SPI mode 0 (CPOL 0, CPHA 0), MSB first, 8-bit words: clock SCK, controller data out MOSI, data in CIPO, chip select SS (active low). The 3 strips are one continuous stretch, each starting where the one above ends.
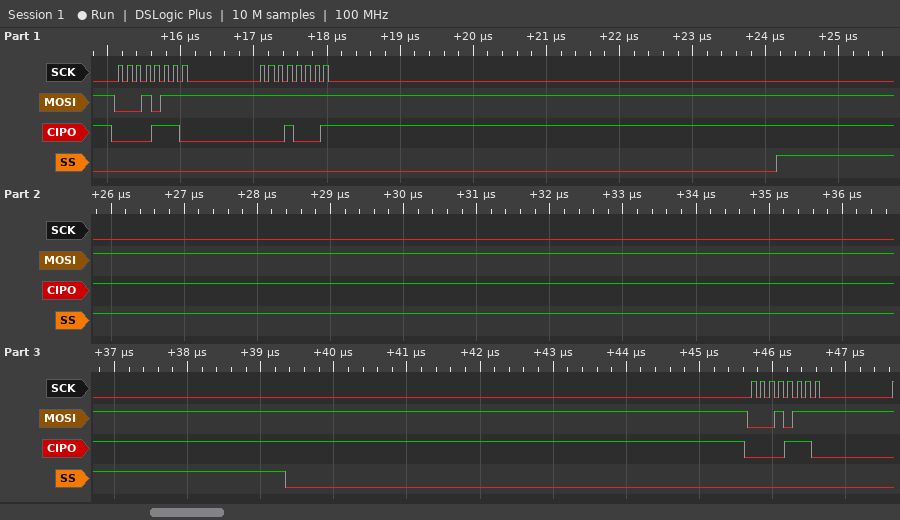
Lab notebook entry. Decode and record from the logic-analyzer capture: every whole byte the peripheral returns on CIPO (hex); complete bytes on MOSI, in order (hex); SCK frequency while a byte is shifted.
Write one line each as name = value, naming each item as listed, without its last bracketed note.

every whole byte the peripheral returns on CIPO = 0x0E 0x11 0x0E
complete bytes on MOSI, in order = 0x17 0xFF 0x17
SCK frequency while a byte is shifted = 8 MHz
